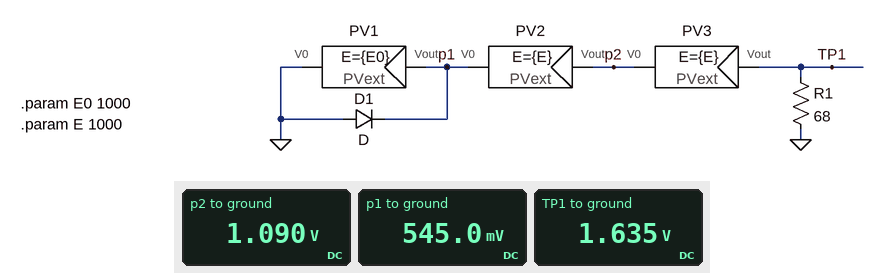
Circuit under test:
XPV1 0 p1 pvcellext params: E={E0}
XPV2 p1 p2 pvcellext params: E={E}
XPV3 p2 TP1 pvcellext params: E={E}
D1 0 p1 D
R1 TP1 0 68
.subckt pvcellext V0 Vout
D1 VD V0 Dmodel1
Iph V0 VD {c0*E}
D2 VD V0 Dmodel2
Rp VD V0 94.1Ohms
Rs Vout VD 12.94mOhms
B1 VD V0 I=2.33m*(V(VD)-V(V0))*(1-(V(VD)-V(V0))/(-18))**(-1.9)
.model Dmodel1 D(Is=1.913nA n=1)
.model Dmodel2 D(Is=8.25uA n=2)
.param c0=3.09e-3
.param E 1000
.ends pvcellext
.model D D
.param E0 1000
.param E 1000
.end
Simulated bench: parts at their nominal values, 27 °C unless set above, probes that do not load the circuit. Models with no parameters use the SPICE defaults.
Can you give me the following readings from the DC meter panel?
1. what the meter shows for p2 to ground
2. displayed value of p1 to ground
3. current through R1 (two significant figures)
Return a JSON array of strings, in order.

["1.090 V", "545.0 mV", "24 mA"]
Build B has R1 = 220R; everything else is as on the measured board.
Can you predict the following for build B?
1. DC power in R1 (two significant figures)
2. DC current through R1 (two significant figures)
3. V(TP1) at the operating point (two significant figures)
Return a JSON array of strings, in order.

["12 mW", "7.4 mA", "1.6 V"]
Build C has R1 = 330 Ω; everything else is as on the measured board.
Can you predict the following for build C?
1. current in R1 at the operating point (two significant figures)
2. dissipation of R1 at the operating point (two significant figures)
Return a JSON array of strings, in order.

["5.0 mA", "8.1 mW"]
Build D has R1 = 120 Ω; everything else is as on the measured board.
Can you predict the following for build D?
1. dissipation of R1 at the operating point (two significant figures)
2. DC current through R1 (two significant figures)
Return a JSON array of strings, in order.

["22 mW", "14 mA"]
